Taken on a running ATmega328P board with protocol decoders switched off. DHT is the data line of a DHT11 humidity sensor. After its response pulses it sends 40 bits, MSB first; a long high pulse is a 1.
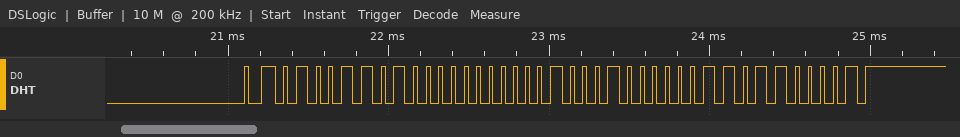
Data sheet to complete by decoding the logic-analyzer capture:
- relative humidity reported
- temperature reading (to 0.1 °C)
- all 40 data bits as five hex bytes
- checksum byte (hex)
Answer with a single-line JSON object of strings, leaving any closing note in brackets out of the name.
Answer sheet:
{"relative humidity reported": "77 %", "temperature reading": "17.3 °C", "all 40 data bits as five hex bytes": "4D 00 11 03 61", "checksum byte": "0x61"}
